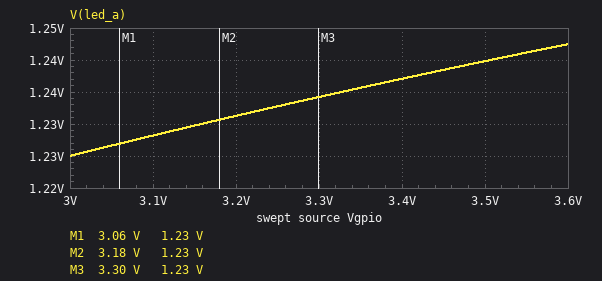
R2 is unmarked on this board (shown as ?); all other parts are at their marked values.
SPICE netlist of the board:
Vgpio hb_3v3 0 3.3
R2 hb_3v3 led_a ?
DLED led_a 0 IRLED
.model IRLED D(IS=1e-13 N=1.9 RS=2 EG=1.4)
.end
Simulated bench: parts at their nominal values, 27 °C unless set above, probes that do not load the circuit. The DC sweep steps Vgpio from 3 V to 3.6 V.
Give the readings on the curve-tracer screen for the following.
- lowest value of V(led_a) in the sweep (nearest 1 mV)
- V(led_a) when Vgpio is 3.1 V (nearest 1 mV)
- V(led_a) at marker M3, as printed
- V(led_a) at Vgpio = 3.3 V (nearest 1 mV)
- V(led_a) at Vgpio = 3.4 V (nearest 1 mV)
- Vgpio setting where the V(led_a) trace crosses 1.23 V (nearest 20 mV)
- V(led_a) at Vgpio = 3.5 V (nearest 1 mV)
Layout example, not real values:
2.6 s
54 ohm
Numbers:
1.225 V
1.228 V
1.23 V
1.234 V
1.237 V
3.16 V
1.240 V
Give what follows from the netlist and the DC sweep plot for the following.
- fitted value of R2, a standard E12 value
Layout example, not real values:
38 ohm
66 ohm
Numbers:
330 Ω
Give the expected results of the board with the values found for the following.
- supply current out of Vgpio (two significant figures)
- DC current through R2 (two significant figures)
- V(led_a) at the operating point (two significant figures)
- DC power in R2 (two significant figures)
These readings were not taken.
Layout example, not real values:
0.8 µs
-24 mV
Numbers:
6.3 mA
6.3 mA
1.2 V
13 mW
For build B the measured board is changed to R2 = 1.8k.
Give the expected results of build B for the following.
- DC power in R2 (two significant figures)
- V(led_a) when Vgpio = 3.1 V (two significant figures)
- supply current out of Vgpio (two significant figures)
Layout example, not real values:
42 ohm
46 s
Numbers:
2.6 mW
1.1 V
1.2 mA
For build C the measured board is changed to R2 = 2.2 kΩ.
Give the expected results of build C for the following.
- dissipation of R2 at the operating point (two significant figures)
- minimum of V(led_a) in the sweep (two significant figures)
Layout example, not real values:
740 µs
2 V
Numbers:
2.1 mW
1.1 V
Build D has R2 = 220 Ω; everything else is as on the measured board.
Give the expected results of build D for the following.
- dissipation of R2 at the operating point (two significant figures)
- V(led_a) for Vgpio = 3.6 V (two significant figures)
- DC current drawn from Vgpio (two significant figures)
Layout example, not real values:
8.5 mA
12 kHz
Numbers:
19 mW
1.3 V
9.3 mA
